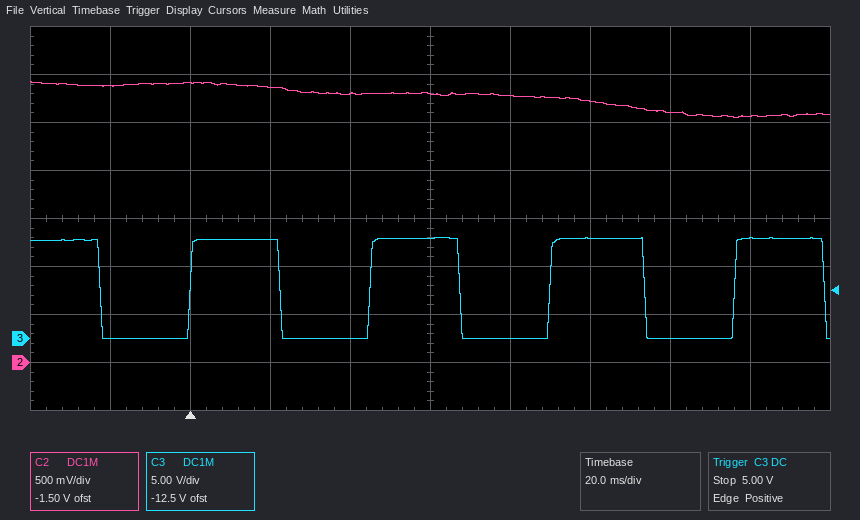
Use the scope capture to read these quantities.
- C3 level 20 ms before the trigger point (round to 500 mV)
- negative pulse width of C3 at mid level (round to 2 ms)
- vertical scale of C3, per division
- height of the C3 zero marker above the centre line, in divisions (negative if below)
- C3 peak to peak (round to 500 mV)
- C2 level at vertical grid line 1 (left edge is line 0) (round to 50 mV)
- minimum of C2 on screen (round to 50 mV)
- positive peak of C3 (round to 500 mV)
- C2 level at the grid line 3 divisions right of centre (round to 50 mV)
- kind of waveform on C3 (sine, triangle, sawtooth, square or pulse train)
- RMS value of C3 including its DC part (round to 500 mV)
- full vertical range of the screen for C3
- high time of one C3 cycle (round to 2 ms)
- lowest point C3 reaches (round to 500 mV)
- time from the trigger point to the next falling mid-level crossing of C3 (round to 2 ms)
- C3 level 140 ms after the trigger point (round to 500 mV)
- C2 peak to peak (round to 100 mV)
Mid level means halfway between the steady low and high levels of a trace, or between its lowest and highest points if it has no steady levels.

0.0 V
22 ms
5 V
-2.5 div
10.5 V
2.90 V
2.55 V
10.5 V
2.60 V
square
7.5 V
40 V
22 ms
0.0 V
22 ms
10.5 V
400 mV
